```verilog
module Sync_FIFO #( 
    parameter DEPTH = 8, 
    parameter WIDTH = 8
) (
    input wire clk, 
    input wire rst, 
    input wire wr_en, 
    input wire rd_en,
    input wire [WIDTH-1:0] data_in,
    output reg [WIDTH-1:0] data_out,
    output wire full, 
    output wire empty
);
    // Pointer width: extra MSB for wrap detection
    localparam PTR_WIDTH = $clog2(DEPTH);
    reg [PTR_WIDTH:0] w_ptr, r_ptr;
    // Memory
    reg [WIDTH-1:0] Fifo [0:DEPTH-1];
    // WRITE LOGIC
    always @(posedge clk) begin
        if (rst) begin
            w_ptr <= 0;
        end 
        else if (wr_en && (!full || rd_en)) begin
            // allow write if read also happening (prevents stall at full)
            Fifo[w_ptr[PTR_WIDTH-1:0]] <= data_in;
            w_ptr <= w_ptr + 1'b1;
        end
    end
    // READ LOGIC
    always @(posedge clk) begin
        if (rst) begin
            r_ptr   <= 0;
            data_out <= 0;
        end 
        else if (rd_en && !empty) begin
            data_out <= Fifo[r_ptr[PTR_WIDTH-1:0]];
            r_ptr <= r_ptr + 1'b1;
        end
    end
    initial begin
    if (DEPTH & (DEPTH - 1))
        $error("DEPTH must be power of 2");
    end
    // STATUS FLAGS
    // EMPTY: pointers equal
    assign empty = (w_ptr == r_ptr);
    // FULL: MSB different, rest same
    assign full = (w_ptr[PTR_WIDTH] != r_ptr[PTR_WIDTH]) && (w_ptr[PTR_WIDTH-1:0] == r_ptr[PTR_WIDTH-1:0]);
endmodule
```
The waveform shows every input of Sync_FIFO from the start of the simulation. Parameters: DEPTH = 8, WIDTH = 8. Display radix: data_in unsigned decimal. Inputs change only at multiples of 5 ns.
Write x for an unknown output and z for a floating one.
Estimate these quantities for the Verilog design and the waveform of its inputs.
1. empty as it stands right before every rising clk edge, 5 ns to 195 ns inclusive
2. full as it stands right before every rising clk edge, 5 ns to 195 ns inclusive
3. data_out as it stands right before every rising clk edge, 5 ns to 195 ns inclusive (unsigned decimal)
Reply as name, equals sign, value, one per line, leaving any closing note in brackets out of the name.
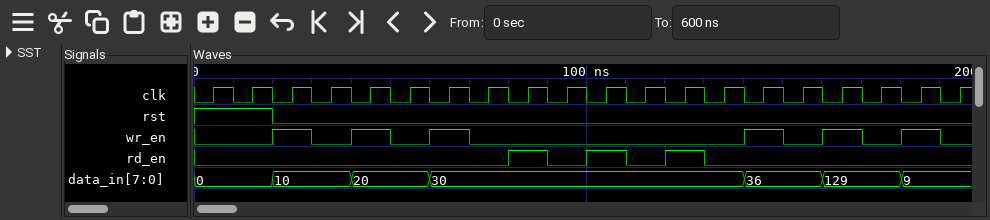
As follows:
empty as it stands right before every rising clk edge, 5 ns to 195 ns inclusive = x 1 1 0 0 0 0 0 0 0 0 0 0 1 1 0 0 0 0 0
full as it stands right before every rising clk edge, 5 ns to 195 ns inclusive = x 0 0 0 0 0 0 0 0 0 0 0 0 0 0 0 0 0 0 0
data_out as it stands right before every rising clk edge, 5 ns to 195 ns inclusive = x, 0, 0, 0, 0, 0, 0, 0, 0, 10, 10, 20, 20, 30, 30, 30, 30, 30, 30, 30
